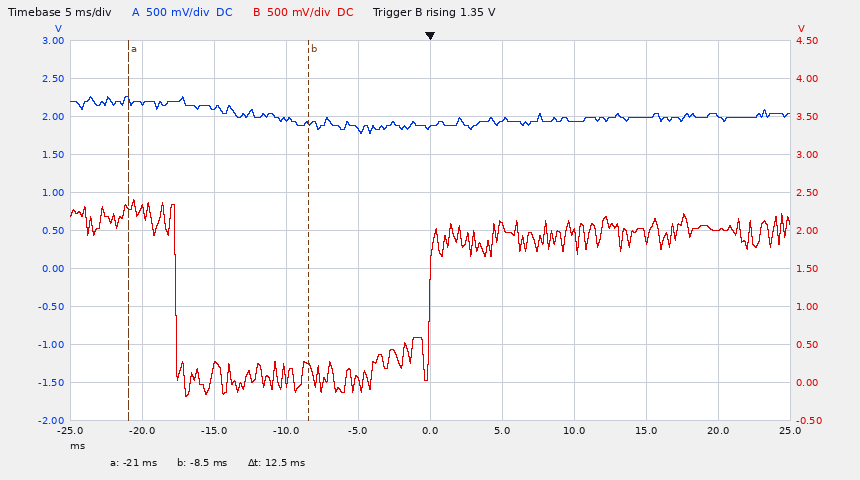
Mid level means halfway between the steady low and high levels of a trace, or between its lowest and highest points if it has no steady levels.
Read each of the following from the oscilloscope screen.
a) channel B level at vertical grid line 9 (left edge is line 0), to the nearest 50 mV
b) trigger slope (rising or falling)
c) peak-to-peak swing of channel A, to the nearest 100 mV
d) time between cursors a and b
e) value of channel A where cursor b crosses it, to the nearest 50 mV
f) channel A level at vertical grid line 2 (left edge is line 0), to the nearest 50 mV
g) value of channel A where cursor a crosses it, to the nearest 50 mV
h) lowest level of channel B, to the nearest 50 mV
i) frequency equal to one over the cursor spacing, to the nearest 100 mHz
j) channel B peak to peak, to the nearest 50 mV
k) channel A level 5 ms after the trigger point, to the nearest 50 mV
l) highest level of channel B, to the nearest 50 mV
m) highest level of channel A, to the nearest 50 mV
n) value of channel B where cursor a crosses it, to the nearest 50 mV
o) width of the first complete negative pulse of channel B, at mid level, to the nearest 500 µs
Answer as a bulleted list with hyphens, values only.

- 2.00 V
- rising
- 500 mV
- 12.5 ms
- 1.90 V
- 2.10 V
- 2.20 V
- -200 mV
- 80.0 Hz
- 2.60 V
- 1.95 V
- 2.40 V
- 2.25 V
- 2.30 V
- 17.5 ms
